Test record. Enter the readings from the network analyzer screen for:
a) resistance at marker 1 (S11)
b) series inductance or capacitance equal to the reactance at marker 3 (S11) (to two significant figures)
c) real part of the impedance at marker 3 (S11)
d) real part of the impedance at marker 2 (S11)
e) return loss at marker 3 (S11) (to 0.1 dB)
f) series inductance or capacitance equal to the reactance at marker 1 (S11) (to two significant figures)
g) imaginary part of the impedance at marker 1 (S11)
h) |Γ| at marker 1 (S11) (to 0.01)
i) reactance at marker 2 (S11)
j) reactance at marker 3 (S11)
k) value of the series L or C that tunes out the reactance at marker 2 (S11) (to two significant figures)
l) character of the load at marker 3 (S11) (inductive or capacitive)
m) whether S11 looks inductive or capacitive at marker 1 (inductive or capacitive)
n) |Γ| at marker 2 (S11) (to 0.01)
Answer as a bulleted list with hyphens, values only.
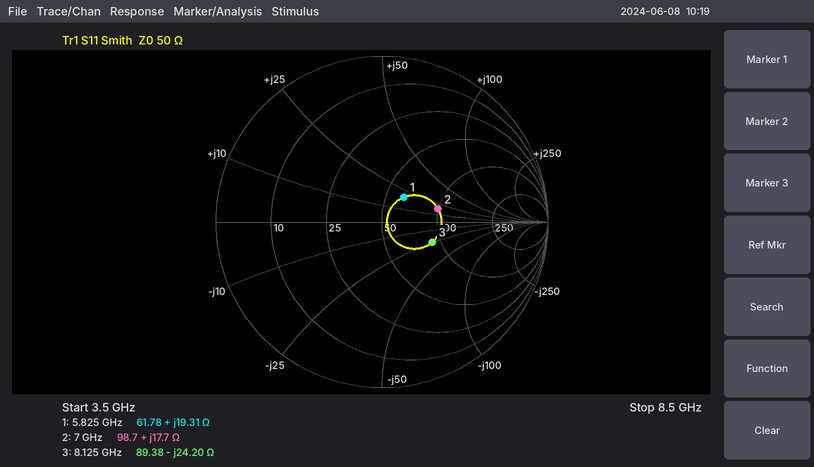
- 61.78 Ω
- 810 fF
- 89.38 Ω
- 98.7 Ω
- 9.7 dB
- 530 pH
- +19.31 Ω
- 0.20
- +17.7 Ω
- -24.20 Ω
- 1.3 pF
- capacitive
- inductive
- 0.35
